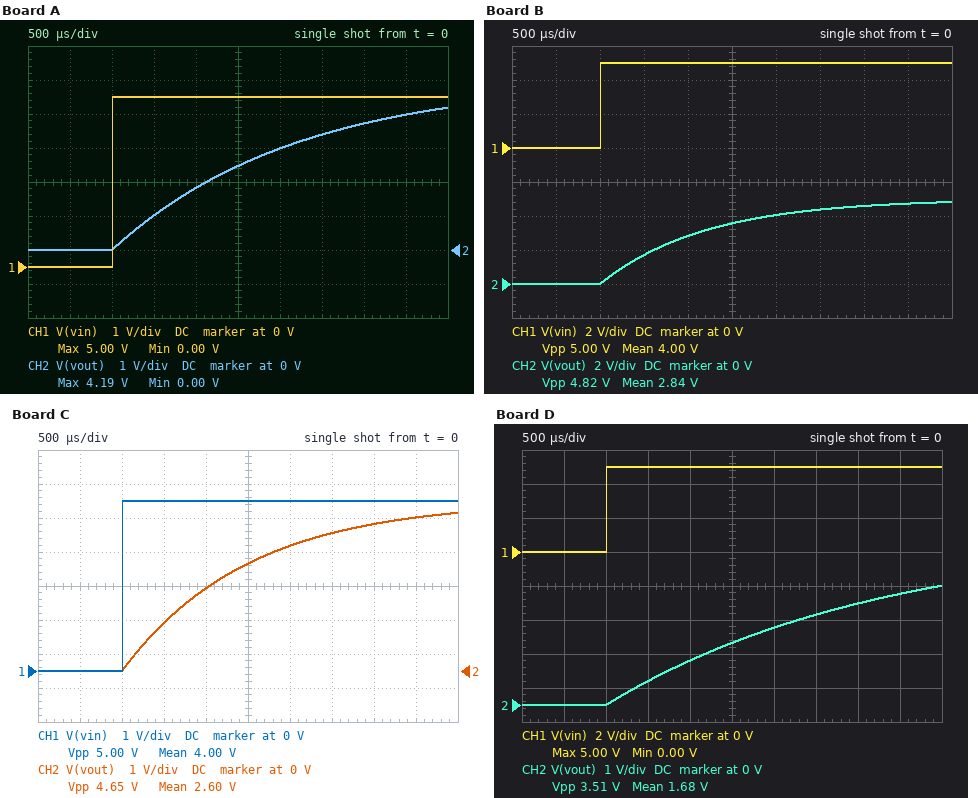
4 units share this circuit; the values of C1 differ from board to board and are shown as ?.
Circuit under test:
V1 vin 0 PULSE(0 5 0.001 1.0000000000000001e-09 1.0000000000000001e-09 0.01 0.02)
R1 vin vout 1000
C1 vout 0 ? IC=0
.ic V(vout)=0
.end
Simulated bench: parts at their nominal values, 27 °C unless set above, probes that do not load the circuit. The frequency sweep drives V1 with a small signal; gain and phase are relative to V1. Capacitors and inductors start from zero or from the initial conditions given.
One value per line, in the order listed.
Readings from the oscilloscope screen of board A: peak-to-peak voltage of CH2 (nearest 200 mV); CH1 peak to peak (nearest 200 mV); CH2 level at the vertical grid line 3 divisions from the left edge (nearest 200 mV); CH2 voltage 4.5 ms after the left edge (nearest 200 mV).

4.2 V
5.0 V
1.0 V
4.0 V
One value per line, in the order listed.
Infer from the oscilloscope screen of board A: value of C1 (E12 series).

2.2 µF
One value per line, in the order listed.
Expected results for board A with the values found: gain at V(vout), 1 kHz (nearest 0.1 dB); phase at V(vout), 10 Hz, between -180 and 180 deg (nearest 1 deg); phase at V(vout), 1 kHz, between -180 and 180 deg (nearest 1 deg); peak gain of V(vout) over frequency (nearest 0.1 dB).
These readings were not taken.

-22.8 dB
-8 deg
-86 deg
0 dB
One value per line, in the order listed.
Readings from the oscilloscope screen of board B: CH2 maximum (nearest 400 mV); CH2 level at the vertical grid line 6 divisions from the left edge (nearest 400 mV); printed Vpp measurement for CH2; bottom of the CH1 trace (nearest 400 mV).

4.8 V
4.0 V
4.82 V
0 V
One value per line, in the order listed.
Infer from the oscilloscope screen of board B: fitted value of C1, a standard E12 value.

1.2 µF
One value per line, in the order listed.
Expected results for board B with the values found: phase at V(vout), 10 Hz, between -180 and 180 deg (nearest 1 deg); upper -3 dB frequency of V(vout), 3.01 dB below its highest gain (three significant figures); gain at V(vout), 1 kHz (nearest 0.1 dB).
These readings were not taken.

-4 deg
133 Hz
-17.6 dB
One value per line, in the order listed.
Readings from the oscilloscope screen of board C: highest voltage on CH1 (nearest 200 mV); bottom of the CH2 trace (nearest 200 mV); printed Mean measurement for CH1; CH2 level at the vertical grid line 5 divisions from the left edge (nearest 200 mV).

5.0 V
0 V
4.00 V
3.2 V
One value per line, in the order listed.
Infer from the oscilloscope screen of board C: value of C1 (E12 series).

1.5 µF
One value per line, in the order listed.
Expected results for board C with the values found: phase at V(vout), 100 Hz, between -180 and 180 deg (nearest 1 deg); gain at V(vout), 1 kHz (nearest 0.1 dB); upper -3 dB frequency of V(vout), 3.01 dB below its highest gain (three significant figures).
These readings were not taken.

-43 deg
-19.5 dB
106 Hz
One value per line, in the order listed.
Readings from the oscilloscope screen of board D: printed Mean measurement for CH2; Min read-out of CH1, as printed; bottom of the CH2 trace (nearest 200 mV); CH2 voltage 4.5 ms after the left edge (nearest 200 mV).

1.68 V
0.00 V
0 V
3.2 V
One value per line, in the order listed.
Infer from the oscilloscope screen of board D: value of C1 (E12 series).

3.3 µF
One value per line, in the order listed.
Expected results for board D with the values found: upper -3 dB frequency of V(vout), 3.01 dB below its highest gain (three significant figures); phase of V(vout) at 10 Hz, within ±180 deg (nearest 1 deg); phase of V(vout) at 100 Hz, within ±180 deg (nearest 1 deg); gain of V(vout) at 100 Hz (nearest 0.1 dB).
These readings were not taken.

48.2 Hz
-12 deg
-64 deg
-7.2 dB
